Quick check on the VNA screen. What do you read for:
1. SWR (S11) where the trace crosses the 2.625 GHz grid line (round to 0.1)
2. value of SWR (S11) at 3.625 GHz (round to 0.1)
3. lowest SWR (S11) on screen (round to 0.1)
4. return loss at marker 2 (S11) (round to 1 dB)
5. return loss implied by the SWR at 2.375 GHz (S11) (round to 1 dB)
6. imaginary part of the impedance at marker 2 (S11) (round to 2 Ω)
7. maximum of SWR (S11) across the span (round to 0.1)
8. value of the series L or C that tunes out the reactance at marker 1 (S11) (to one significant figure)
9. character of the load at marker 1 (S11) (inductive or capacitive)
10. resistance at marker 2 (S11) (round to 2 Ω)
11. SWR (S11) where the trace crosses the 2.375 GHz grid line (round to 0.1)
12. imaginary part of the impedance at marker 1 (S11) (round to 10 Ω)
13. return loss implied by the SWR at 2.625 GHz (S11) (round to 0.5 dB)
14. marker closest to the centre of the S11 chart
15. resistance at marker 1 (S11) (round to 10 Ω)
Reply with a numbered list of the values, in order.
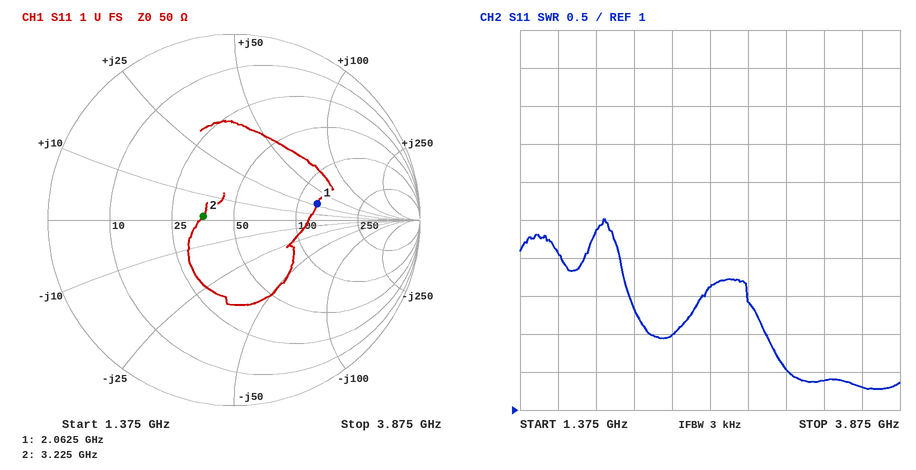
1. 2.6
2. 1.3
3. 1.3
4. 16 dB
5. 10 dB
6. +2 Ω
7. 3.5
8. 3 pF
9. inductive
10. 36 Ω
11. 2.0
12. +30 Ω
13. 7.0 dB
14. marker 2
15. 130 Ω
